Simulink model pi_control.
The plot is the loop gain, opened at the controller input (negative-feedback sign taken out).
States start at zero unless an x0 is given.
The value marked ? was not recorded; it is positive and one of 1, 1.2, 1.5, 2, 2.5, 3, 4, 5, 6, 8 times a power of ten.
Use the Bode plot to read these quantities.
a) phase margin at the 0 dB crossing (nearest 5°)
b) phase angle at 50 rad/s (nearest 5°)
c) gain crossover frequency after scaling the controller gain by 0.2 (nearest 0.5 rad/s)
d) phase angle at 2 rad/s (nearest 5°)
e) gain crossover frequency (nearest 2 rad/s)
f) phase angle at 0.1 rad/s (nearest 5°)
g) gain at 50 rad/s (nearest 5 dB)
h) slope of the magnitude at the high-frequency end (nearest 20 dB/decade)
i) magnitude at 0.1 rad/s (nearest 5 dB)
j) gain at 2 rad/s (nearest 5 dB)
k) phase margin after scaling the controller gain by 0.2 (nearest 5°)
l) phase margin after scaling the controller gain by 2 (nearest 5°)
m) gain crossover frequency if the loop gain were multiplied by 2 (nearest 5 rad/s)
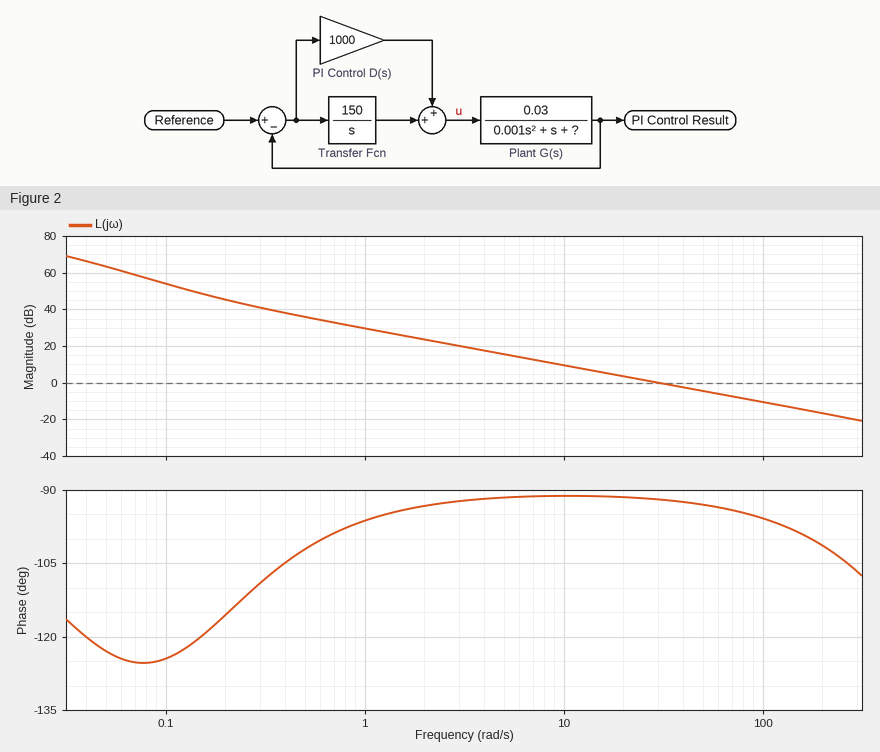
90°
-95°
6.0 rad/s
-95°
30 rad/s
-125°
-5 dB
-20 dB/decade
55 dB
25 dB
90°
85°
60 rad/s
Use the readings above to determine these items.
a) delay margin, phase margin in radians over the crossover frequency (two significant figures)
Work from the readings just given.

0.052 s
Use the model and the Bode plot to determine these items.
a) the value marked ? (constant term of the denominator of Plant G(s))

0.04
